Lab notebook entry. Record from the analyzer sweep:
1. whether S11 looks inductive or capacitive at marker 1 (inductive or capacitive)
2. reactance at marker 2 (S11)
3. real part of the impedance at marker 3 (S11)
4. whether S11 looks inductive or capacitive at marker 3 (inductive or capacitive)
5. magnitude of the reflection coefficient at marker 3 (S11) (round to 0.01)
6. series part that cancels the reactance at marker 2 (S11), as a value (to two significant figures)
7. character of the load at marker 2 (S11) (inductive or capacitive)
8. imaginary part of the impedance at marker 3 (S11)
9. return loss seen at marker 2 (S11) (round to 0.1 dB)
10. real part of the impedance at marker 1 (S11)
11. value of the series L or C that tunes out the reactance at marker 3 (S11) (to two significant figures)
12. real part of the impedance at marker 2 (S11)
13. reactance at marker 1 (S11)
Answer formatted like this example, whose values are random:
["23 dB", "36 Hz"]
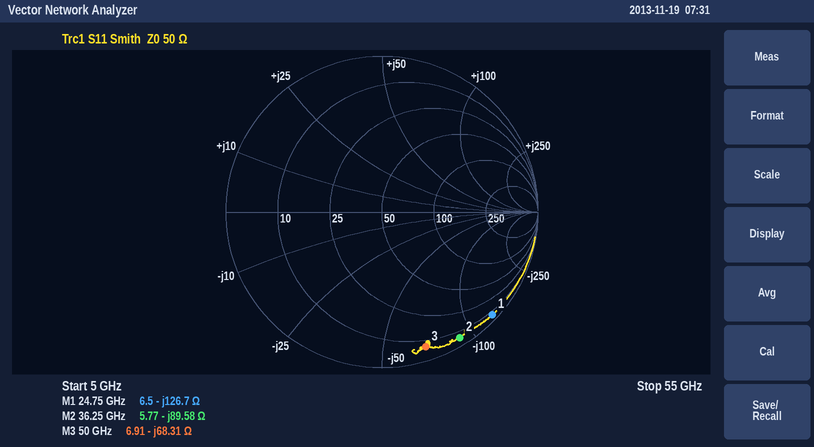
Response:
["capacitive", "-89.58 Ω", "6.91 Ω", "capacitive", "0.91", "390 pH", "capacitive", "-68.31 Ω", "0.5 dB", "6.5 Ω", "220 pH", "5.77 Ω", "-126.7 Ω"]
